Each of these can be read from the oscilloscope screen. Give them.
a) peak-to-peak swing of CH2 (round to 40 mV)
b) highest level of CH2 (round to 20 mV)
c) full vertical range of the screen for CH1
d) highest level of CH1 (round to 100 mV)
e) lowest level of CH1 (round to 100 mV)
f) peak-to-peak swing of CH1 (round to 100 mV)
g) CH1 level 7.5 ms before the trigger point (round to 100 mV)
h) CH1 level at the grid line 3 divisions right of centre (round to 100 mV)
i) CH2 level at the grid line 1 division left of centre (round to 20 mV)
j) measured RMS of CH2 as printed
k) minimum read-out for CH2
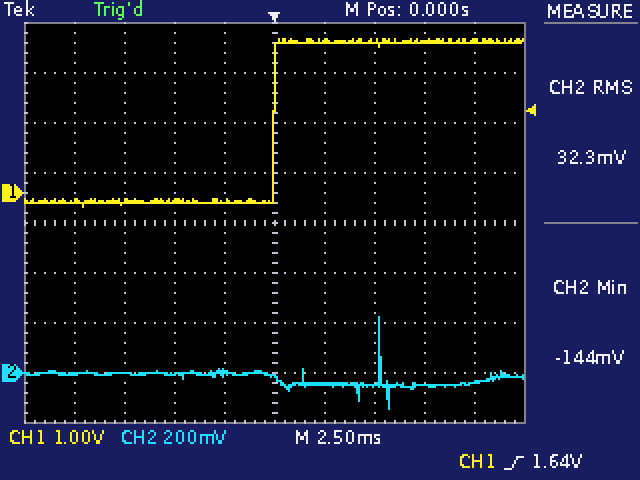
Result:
360 mV
220 mV
8 V
3.1 V
-300 mV
3.4 V
-200 mV
3.0 V
0 mV
32.3 mV
-144 mV
